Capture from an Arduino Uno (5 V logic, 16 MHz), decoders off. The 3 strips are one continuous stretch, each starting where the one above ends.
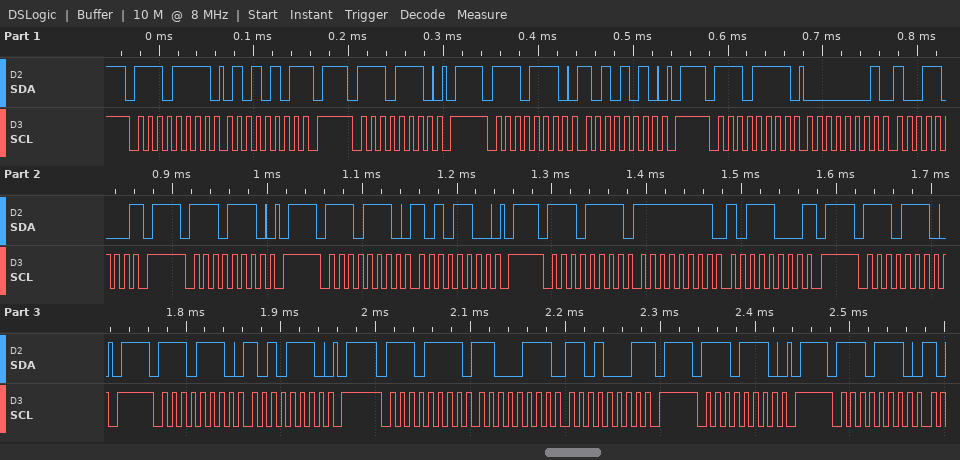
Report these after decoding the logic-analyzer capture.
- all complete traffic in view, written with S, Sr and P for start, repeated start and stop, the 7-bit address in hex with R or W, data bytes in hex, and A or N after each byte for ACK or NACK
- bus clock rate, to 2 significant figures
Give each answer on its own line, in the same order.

S 77R A 55 N P S 77W A P S 77W A AA A P S 77R A 01 A 98 N P S 77W A P S 77W A AC A P S 77R A FF A B8 N P S 77W A P S 77W A AE A P S 77R A C7 A D1 N P S 77W A P S 77W A
100 kHz
